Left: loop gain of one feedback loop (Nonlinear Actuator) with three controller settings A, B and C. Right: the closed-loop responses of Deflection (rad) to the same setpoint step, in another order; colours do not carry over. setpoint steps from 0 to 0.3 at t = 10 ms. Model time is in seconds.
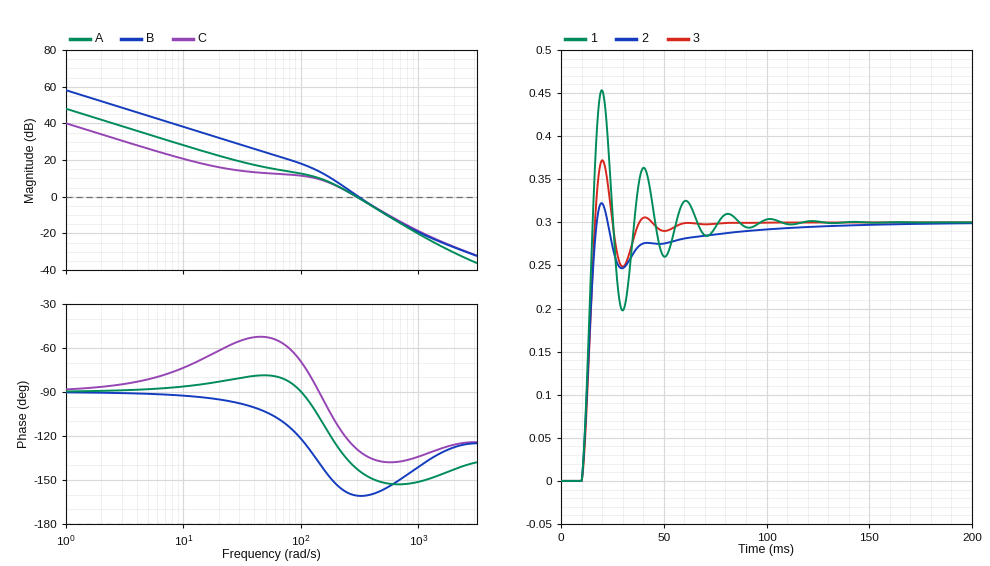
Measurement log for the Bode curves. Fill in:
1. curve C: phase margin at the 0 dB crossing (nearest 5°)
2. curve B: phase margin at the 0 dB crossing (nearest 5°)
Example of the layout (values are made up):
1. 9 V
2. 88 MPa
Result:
1. 50°
2. 20°
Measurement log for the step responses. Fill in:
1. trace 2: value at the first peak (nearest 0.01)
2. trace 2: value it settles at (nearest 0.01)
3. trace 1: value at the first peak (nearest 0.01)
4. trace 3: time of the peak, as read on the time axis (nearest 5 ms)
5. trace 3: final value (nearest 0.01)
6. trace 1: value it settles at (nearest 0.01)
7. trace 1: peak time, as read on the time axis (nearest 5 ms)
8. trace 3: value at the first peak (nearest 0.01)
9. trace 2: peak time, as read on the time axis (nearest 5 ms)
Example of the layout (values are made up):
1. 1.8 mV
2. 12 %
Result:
1. 0.32
2. 0.30
3. 0.45
4. 20 ms
5. 0.30
6. 0.30
7. 20 ms
8. 0.37
9. 20 ms
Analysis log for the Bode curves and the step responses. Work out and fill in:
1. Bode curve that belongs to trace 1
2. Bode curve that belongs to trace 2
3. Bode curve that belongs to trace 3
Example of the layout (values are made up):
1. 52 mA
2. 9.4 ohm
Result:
1. B
2. C
3. A
